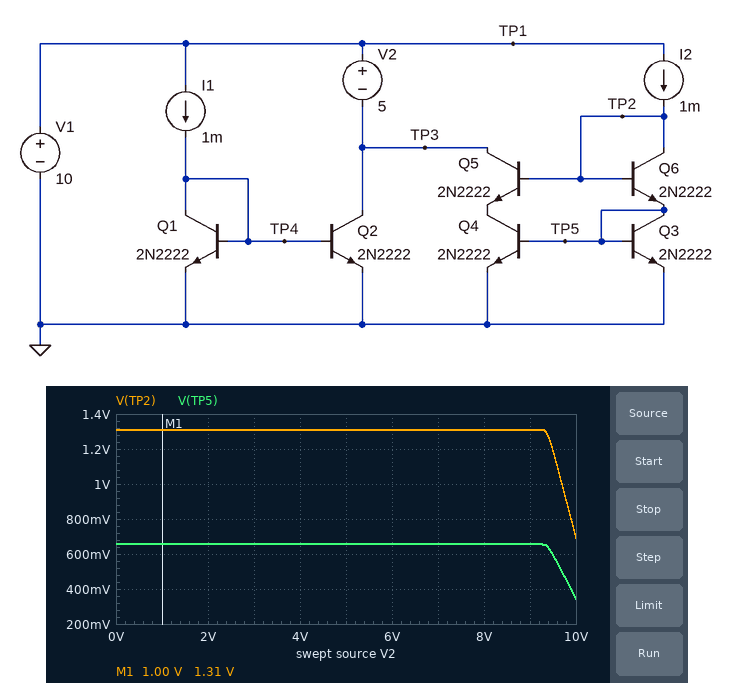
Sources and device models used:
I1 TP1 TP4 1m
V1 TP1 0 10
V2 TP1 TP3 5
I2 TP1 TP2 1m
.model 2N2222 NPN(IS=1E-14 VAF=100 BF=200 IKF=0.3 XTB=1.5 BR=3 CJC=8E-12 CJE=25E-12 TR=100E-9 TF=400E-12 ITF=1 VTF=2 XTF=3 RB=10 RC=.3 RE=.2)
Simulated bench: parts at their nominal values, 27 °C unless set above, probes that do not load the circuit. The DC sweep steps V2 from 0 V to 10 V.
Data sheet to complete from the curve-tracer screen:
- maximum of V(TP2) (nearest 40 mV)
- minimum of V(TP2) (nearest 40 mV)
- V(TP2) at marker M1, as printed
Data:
1.32 V
680 mV
1.31 V
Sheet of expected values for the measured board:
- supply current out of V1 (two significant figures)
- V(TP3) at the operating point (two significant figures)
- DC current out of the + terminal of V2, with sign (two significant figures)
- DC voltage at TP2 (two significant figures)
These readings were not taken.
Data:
4.0 mA
5.0 V
-2.0 mA
1.3 V
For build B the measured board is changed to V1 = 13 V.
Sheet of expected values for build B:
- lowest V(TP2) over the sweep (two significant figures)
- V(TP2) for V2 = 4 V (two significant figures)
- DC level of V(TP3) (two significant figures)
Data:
1.3 V
1.3 V
8.0 V
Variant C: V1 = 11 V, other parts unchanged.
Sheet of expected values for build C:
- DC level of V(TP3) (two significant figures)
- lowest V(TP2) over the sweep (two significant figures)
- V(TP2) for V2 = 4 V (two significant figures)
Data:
6.0 V
1.3 V
1.3 V
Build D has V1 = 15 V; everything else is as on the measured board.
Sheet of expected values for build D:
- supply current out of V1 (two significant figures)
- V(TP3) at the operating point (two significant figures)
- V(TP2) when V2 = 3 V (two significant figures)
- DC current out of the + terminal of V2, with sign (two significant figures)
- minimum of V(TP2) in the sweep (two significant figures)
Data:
4.1 mA
10 V
1.3 V
-2.1 mA
1.3 V
